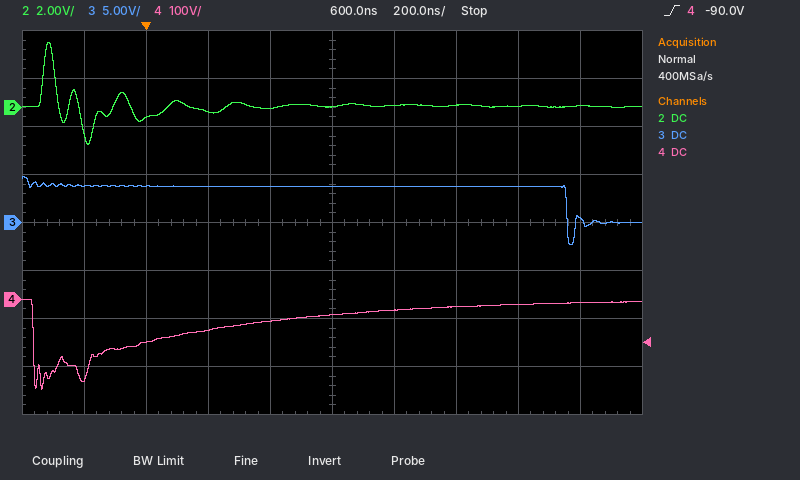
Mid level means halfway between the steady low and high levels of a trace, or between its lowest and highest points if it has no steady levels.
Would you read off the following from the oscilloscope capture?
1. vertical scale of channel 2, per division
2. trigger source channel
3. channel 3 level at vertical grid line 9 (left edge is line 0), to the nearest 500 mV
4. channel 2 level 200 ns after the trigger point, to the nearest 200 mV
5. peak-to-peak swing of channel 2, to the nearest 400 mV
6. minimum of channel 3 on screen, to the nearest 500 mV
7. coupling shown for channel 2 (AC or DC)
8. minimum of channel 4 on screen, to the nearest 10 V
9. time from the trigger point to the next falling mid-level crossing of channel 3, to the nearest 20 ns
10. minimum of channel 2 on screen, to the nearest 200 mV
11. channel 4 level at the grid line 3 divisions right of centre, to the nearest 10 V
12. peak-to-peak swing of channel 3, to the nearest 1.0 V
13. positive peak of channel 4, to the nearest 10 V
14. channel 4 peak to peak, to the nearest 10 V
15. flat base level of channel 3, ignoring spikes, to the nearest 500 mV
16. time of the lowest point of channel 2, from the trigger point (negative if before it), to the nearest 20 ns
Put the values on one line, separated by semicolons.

2 V; channel 4; 500 mV; -200 mV; 4.4 V; -2.5 V; DC; -190 V; 1.36 µs; -1.6 V; -10 V; 7.0 V; 0 V; 190 V; 0.0 V; -180 ns
